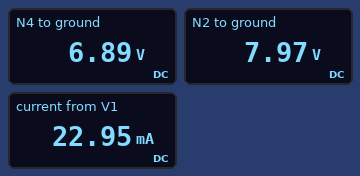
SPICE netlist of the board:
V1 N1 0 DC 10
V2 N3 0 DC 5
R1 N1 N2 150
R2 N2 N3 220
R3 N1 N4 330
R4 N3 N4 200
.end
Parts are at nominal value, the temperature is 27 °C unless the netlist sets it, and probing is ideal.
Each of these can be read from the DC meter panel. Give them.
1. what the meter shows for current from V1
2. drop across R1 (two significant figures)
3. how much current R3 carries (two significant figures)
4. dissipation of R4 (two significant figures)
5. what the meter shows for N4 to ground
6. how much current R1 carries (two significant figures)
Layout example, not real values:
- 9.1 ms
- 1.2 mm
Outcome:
- 22.95 mA
- 2.0 V
- 9.4 mA
- 18 mW
- 6.89 V
- 14 mA
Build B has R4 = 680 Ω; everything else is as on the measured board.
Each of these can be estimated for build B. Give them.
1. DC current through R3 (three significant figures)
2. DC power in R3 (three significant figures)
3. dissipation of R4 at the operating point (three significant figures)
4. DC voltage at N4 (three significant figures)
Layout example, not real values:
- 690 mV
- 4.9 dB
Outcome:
- 4.95 mA
- 8.09 mW
- 16.7 mW
- 8.37 V
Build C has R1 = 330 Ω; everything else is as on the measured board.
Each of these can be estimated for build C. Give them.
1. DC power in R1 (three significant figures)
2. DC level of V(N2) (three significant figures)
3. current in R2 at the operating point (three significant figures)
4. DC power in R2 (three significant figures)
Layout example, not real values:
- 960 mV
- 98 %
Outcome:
- 27.3 mW
- 7.00 V
- 9.09 mA
- 18.2 mW
